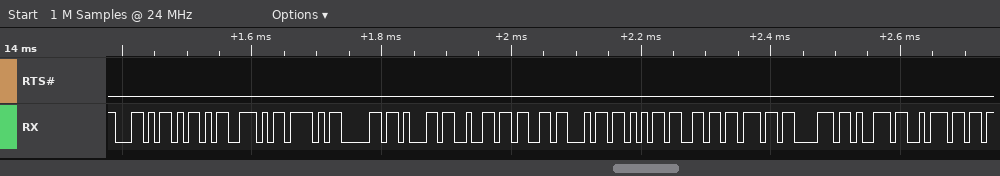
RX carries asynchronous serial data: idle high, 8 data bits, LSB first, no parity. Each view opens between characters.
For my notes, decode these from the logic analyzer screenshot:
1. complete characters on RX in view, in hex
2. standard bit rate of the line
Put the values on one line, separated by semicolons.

AC, AD, AE, AF, B0, B1, B2, B3, B4, B5, B6, B7, B8, B9, BA; 115200 baud
